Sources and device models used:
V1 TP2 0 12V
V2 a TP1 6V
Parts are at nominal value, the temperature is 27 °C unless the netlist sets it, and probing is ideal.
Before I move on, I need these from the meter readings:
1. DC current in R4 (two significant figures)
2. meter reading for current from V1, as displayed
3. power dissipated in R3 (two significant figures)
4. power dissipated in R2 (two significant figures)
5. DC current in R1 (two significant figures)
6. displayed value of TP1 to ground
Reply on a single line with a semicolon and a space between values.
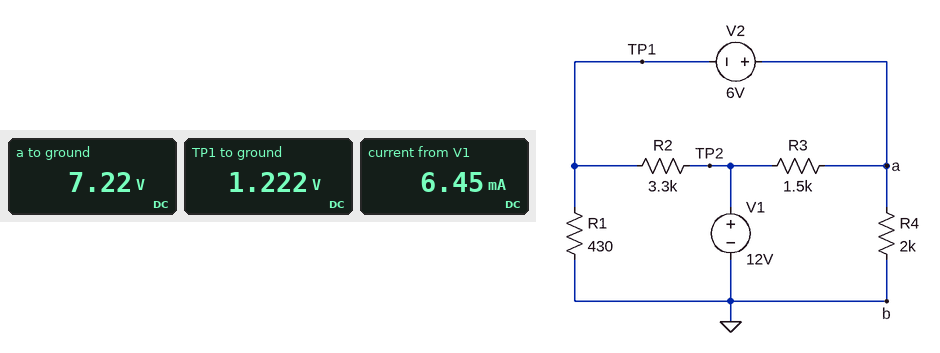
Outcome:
3.6 mA; 6.45 mA; 15 mW; 35 mW; 2.8 mA; 1.222 V
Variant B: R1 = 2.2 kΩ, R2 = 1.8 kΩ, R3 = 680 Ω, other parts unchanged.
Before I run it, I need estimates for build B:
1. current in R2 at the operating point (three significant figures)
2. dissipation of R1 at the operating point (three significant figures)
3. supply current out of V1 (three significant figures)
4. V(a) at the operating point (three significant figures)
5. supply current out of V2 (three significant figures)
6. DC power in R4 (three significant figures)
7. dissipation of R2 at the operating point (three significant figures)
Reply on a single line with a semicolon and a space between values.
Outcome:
4.34 mA; 7.98 mW; 7.00 mA; 10.2 V; 2.43 mA; 51.9 mW; 33.9 mW
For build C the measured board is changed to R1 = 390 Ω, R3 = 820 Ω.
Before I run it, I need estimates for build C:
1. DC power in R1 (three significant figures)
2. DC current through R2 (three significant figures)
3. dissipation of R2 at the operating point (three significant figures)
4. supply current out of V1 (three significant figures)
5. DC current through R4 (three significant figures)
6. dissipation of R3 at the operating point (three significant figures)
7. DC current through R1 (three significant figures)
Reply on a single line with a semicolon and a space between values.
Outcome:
7.71 mW; 3.11 mA; 31.9 mW; 8.31 mA; 3.87 mA; 22.2 mW; 4.45 mA
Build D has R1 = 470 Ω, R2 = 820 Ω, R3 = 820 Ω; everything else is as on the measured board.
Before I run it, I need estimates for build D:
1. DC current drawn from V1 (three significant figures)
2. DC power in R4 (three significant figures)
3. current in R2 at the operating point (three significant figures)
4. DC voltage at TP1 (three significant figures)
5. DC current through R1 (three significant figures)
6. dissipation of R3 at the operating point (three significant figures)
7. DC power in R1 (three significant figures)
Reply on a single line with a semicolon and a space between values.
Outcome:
12.8 mA; 47.4 mW; 10.1 mA; 3.74 V; 7.96 mA; 6.23 mW; 29.8 mW
